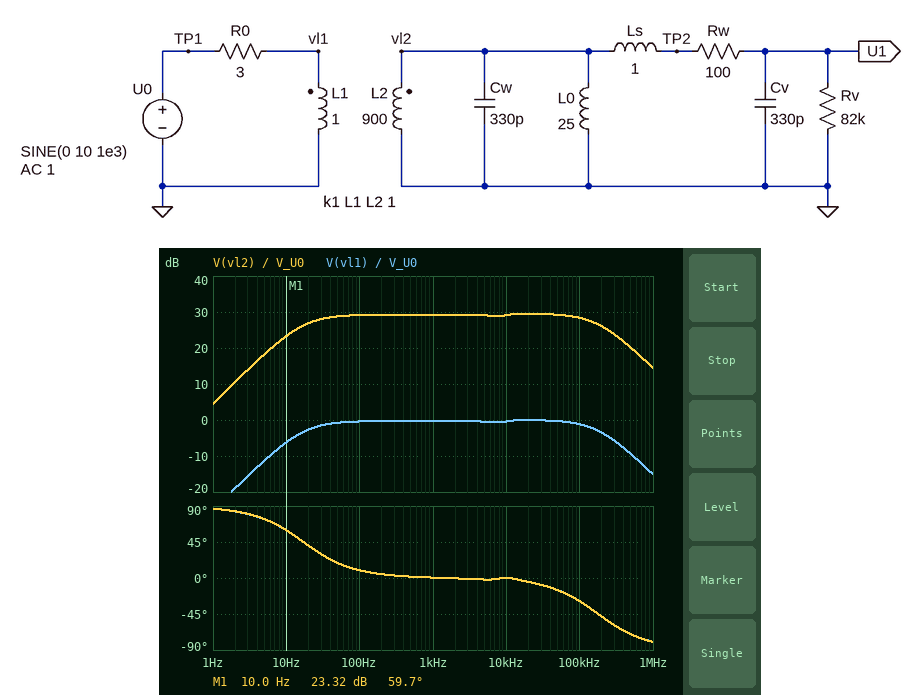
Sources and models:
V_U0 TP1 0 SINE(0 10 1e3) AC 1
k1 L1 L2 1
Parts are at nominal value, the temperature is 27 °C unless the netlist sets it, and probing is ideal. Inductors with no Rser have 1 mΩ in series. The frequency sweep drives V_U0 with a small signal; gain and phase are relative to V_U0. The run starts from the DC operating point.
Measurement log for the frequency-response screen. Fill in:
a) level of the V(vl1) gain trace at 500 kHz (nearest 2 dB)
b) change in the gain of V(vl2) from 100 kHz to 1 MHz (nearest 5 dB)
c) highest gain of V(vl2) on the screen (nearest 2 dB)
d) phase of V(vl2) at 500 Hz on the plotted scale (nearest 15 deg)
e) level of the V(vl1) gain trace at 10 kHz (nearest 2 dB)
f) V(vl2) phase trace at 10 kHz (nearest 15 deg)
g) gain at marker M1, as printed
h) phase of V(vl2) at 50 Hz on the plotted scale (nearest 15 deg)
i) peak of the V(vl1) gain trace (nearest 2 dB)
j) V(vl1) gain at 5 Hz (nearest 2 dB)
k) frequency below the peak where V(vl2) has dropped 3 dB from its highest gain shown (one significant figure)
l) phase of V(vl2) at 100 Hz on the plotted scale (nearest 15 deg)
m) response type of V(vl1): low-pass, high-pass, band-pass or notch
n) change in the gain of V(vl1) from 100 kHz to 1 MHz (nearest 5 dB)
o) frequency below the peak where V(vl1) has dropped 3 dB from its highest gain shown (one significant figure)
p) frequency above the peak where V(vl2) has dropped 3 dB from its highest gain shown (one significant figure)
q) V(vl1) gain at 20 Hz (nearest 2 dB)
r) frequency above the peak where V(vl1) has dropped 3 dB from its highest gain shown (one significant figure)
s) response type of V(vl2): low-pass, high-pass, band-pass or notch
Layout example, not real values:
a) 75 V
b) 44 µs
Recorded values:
a) -10 dB
b) -15 dB
c) 30 dB
d) 0 deg
e) 0 dB
f) 0 deg
g) 23.32 dB
h) 15 deg
i) 0 dB
j) -12 dB
k) 20 Hz
l) 15 deg
m) band-pass
n) -15 dB
o) 20 Hz
p) 200 kHz
q) -2 dB
r) 200 kHz
s) band-pass
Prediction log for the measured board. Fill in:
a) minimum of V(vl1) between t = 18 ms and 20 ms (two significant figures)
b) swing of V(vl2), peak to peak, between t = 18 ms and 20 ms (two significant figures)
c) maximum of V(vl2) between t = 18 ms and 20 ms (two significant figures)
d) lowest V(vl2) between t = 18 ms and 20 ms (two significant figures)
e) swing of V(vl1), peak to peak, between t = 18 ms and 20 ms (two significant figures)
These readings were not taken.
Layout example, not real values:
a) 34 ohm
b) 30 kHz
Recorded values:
a) -9.7 V
b) 580 V
c) 290 V
d) -290 V
e) 19 V
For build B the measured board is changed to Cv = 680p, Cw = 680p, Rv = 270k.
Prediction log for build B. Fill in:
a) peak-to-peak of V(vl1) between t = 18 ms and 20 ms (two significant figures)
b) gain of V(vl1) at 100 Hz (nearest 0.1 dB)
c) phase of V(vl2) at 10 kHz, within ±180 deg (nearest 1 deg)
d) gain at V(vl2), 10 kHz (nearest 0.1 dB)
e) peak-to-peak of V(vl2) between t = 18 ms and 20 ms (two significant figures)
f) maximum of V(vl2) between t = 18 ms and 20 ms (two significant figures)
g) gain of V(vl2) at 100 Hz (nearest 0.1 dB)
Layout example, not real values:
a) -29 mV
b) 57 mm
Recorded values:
a) 20 V
b) -0.2 dB
c) -3 deg
d) 29.5 dB
e) 590 V
f) 300 V
g) 29.3 dB
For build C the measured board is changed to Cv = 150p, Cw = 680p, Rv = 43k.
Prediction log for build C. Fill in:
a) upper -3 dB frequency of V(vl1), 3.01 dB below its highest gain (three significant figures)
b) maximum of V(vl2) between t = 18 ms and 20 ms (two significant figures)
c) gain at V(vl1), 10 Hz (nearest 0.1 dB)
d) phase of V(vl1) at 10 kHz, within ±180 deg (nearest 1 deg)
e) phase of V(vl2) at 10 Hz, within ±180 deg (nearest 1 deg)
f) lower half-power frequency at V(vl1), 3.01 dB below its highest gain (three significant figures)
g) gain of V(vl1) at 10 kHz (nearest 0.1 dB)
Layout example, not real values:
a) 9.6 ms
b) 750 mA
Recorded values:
a) 91.0 kHz
b) 280 V
c) -6.3 dB
d) -4 deg
e) 59 deg
f) 18.0 Hz
g) -0.3 dB
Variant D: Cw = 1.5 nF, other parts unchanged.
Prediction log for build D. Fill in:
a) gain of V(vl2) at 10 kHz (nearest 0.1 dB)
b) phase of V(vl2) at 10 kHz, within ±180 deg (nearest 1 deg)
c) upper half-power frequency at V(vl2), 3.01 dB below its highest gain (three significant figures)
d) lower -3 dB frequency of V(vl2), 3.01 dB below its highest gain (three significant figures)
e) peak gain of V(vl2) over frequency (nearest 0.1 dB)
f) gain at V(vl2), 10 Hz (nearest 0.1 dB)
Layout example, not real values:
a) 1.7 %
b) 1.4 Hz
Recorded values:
a) 29.0 dB
b) -10 deg
c) 42.3 kHz
d) 17.1 Hz
e) 29.3 dB
f) 23.3 dB
